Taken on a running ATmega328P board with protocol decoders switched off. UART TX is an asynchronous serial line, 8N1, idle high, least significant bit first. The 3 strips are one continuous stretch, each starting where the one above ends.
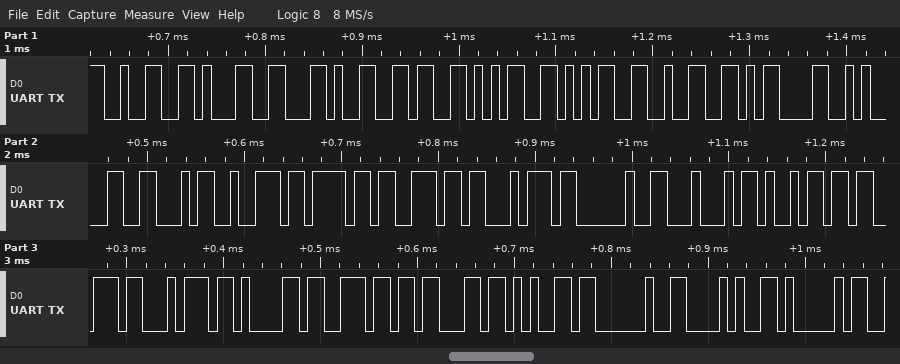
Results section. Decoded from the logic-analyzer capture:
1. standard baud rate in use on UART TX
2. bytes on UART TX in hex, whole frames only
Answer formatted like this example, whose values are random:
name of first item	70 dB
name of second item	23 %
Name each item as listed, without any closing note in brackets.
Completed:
standard baud rate in use on UART TX	115200 baud
bytes on UART TX in hex, whole frames only	32 31 2C 36 35 35 32 0D 0A 46 72 6F 6E 74 20 44 69 73 74 61 6E 63 65 20 28 41
